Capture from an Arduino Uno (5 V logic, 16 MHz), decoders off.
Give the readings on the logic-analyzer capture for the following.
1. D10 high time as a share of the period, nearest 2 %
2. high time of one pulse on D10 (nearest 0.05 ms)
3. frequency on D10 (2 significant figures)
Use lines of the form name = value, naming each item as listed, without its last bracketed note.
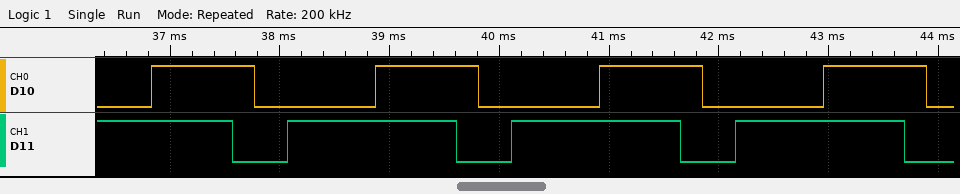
D10 high time as a share of the period, nearest 2 % = 46 %
high time of one pulse on D10 = 0.95 ms
frequency on D10 = 490 Hz
